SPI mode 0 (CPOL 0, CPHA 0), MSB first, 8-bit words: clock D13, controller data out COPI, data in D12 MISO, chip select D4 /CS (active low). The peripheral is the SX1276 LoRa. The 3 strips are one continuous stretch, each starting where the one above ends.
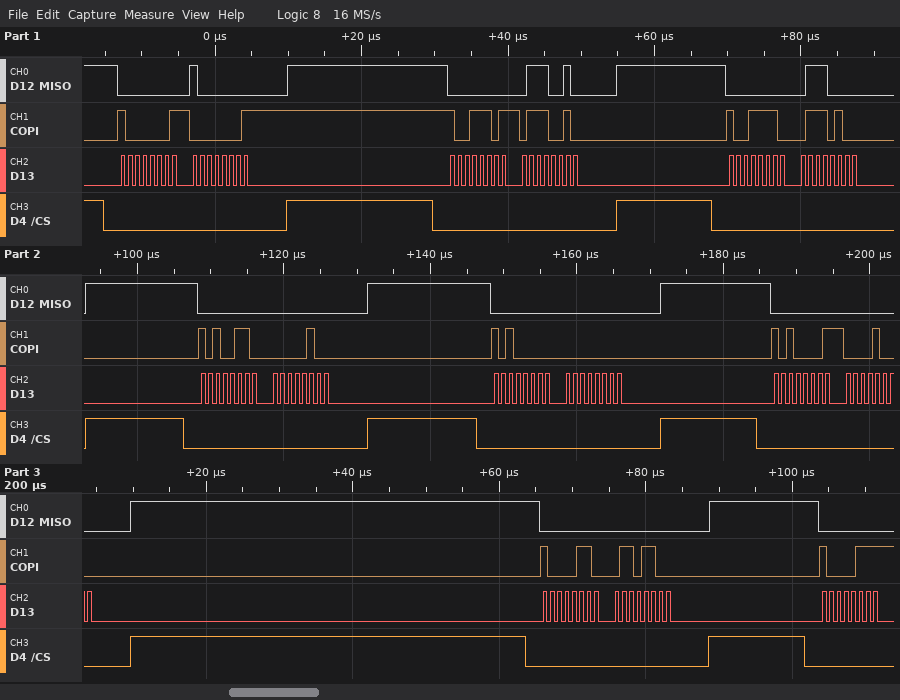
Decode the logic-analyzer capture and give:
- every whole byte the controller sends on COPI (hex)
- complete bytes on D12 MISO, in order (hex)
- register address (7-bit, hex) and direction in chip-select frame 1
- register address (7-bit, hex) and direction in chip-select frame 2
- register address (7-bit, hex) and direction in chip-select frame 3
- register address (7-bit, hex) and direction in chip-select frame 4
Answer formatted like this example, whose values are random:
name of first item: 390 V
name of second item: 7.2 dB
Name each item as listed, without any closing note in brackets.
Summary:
every whole byte the controller sends on COPI: 81 01 9D 72 9E 74 A6 04 A0 00 A1 08 86 6C 87
complete bytes on D12 MISO, in order: 00 80 00 72 00 70 00 00 00 00 00 00 00 00 00
register address (7-bit, hex) and direction in chip-select frame 1: 0x01 write
register address (7-bit, hex) and direction in chip-select frame 2: 0x1D write
register address (7-bit, hex) and direction in chip-select frame 3: 0x1E write
register address (7-bit, hex) and direction in chip-select frame 4: 0x26 write
